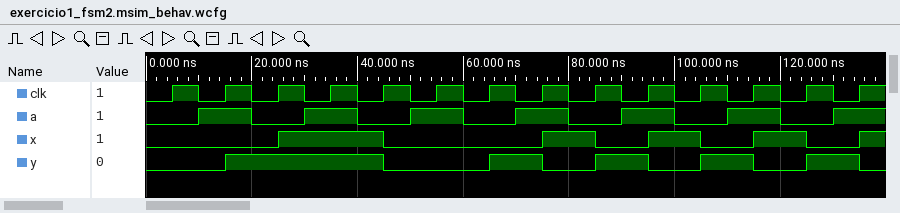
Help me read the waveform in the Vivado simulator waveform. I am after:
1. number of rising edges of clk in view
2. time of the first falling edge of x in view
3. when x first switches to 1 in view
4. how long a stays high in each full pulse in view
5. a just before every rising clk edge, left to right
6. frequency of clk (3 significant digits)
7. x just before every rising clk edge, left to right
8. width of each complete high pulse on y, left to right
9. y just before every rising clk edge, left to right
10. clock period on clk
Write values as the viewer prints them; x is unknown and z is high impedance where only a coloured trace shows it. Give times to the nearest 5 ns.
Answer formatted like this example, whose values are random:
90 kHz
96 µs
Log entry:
14
45 ns
25 ns
10 ns, 10 ns, 10 ns, 10 ns, 10 ns, 10 ns
0 1 0 1 0 1 0 1 0 1 0 1 0 1
100 MHz
0 0 0 1 1 0 0 0 1 0 1 0 1 0
30 ns, 10 ns, 10 ns, 10 ns, 10 ns
0 0 1 1 1 0 0 1 0 1 0 1 0 1
10 ns
